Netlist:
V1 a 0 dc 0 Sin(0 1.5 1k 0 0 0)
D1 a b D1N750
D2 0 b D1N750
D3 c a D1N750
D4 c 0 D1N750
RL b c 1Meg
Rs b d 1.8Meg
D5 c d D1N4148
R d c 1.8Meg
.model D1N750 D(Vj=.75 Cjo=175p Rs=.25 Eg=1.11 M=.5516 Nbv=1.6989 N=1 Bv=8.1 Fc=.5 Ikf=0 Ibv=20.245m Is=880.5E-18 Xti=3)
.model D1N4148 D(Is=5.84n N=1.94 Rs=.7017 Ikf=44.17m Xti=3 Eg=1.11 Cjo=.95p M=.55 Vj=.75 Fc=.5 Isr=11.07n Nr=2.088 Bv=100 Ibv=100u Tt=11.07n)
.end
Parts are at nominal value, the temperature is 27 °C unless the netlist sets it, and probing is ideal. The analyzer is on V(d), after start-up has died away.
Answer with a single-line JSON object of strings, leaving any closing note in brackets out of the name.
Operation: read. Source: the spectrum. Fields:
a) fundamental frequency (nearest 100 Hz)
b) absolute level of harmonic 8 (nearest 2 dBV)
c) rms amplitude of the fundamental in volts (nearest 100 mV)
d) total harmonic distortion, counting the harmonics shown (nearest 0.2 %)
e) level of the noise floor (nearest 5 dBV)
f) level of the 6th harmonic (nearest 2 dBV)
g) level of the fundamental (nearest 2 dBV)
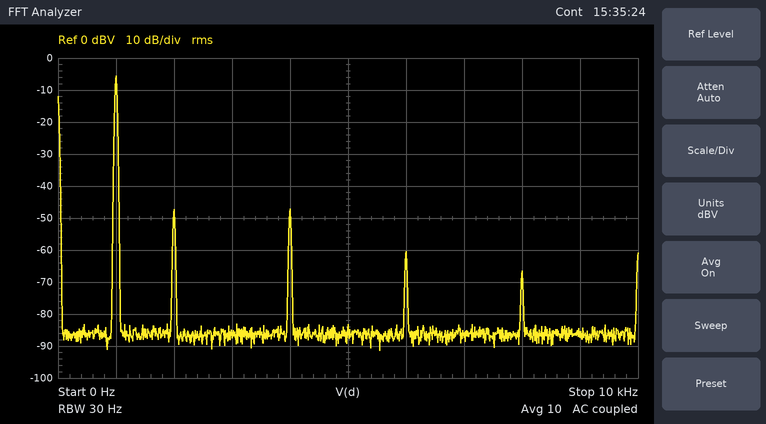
{"fundamental frequency": "1.0 kHz", "absolute level of harmonic 8": "-66 dBV", "rms amplitude of the fundamental in volts": "500 mV", "total harmonic distortion, counting the harmonics shown": "1.2 %", "level of the noise floor": "-85 dBV", "level of the 6th harmonic": "-60 dBV", "level of the fundamental": "-6 dBV"}
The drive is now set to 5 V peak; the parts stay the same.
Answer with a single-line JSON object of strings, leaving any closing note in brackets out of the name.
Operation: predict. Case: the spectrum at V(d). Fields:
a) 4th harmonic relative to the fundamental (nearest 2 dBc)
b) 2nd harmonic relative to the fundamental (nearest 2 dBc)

{"4th harmonic relative to the fundamental": "-60 dBc", "2nd harmonic relative to the fundamental": "-52 dBc"}
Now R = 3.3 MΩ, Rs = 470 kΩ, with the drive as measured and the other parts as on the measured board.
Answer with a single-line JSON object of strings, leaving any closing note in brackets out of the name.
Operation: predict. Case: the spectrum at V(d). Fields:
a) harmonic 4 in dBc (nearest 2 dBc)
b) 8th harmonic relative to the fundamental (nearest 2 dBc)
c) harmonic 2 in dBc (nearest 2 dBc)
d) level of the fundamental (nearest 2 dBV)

{"harmonic 4 in dBc": "-34 dBc", "8th harmonic relative to the fundamental": "-52 dBc", "harmonic 2 in dBc": "-18 dBc", "level of the fundamental": "-6 dBV"}
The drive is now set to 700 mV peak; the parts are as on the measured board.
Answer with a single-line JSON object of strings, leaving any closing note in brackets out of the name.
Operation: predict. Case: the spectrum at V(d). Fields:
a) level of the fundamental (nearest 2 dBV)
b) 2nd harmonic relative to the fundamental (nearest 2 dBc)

{"level of the fundamental": "-12 dBV", "2nd harmonic relative to the fundamental": "-38 dBc"}
